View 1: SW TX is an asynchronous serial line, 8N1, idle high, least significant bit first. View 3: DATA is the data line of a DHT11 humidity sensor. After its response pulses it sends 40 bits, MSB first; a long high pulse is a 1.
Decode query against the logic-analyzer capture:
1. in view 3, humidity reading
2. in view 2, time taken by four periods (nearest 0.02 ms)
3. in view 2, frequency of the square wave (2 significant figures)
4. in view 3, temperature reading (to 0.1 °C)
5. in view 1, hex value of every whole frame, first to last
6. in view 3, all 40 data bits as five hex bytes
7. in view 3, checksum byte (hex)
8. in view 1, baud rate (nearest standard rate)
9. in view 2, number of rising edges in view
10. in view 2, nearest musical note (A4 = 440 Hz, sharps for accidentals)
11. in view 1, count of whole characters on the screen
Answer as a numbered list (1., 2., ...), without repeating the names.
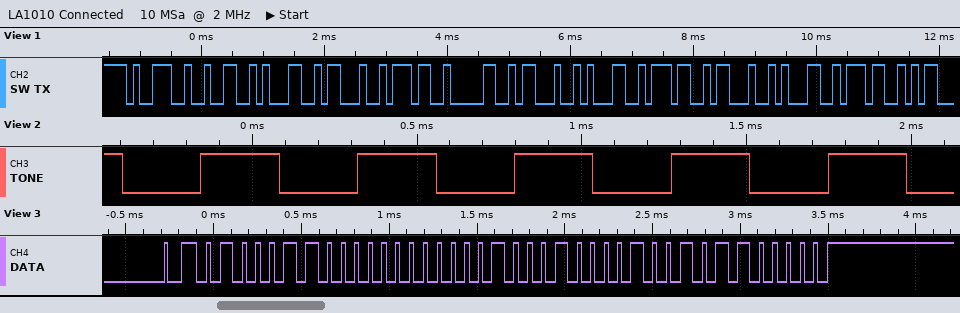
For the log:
1. 70 %
2. 1.90 ms
3. 2.1 kHz
4. 17.9 °C
5. 39 32 31 23 37 30 23 31 37 23 31 37
6. 46 00 11 09 60
7. 0x60
8. 9600 baud
9. 5
10. C7
11. 12
